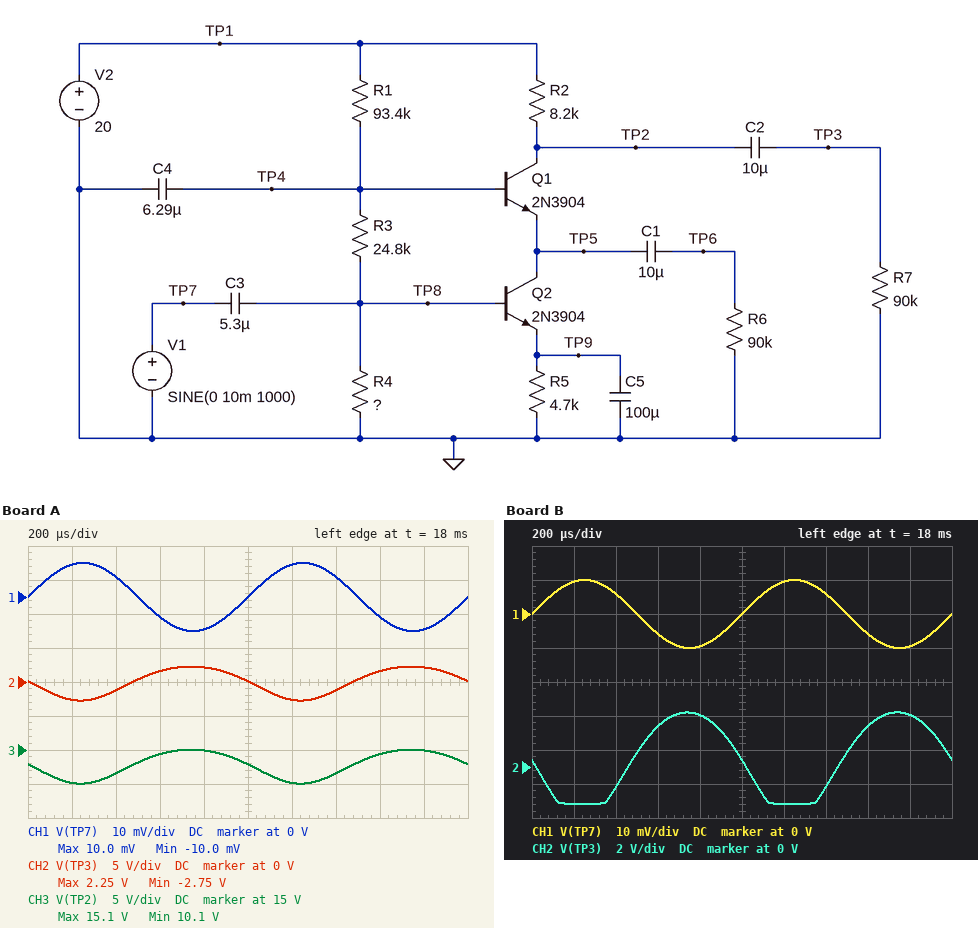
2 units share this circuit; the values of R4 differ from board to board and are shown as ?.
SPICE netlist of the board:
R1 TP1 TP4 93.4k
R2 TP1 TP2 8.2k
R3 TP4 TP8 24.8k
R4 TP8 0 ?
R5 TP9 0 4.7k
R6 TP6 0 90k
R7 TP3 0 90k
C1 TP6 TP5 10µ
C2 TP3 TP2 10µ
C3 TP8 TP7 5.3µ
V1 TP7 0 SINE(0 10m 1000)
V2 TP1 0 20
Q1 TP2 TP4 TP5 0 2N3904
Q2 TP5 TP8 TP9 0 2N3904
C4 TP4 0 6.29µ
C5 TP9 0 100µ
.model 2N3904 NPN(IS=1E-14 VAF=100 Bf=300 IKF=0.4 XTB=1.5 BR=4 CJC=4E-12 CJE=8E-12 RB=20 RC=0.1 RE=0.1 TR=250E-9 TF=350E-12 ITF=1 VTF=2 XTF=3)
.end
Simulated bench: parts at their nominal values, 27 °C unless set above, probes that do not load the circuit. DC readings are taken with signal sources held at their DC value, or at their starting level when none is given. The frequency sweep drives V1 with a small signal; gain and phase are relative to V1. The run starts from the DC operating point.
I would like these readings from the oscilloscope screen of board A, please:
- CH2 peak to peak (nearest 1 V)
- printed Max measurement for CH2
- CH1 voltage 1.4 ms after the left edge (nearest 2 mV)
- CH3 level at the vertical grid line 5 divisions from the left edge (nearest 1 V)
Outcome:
5 V
2.25 V
6 mV
13 V
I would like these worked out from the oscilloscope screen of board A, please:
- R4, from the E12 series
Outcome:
39 kΩ
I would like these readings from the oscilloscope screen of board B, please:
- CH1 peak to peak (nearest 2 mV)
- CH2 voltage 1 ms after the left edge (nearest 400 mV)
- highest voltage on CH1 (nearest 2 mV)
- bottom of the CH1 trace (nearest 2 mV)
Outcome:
20 mV
400 mV
10 mV
-10 mV
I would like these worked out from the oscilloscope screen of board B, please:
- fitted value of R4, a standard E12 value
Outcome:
56 kΩ
